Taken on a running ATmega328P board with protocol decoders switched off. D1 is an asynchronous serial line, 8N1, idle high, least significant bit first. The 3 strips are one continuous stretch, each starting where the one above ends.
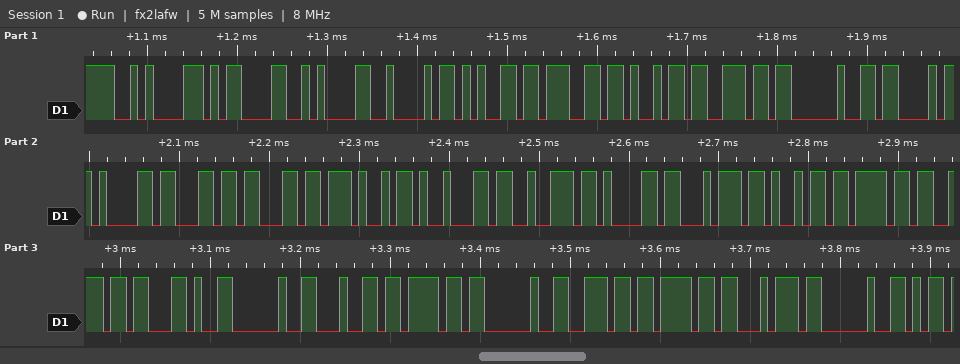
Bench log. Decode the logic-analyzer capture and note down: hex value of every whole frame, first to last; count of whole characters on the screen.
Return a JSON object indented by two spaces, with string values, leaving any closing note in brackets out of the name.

{
  "hex value of every whole frame, first to last": "0A 0D 0A 42 65 67 69 6E 20 43 61 6C 6C 69 62 72 61 74 69 6F 6E 2C 20 64 6F 20 6E 6F 74 20",
  "count of whole characters on the screen": "30"
}
